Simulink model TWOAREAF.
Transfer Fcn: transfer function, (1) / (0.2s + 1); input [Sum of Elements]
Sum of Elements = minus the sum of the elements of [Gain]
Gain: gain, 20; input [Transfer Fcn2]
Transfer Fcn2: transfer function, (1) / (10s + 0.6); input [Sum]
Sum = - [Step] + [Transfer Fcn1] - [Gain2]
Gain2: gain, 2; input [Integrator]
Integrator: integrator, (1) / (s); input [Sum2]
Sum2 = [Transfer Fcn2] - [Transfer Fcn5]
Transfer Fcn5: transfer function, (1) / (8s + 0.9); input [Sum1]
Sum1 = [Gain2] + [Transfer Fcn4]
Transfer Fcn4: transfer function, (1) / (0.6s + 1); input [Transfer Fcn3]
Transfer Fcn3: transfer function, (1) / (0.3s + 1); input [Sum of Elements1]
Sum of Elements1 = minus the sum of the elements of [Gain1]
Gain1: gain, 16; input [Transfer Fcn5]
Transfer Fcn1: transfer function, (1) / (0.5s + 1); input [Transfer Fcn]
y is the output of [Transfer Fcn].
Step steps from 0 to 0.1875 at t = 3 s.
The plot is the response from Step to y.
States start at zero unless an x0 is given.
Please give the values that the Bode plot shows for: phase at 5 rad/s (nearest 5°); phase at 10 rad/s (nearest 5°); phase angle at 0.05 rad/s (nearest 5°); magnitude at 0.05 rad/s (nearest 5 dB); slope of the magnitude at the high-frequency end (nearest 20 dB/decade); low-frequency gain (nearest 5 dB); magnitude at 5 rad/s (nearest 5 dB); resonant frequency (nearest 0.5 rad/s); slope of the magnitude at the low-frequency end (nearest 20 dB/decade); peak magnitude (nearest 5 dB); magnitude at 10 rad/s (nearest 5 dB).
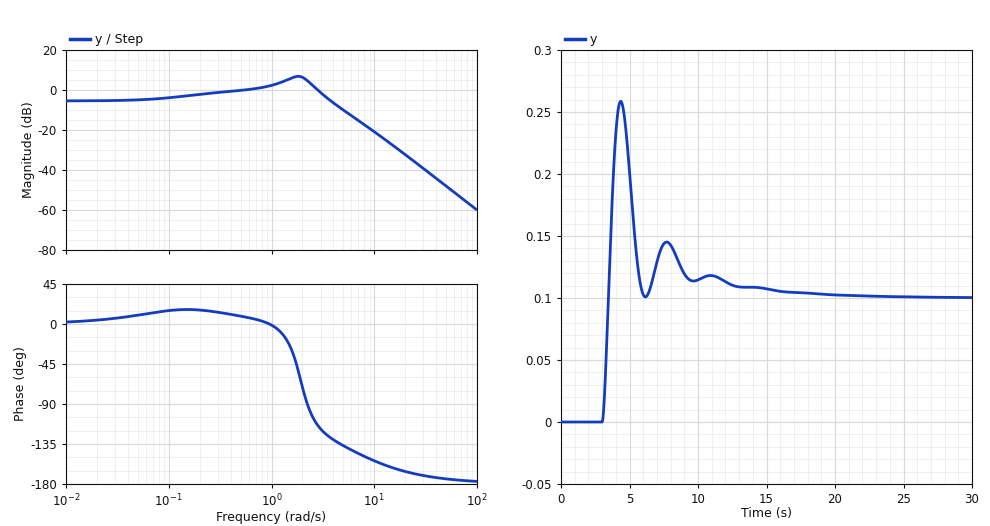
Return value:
-135°
-155°
10°
-5 dB
-40 dB/decade
-5 dB
-10 dB
2.0 rad/s
0 dB/decade
5 dB
-20 dB
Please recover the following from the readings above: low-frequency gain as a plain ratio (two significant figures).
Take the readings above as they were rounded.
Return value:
0.56
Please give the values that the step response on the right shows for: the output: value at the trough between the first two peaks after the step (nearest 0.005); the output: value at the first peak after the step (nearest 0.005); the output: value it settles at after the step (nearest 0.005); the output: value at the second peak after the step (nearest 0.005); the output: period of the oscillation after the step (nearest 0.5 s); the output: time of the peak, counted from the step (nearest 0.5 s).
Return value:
0.100
0.260
0.100
0.145
3.5 s
1.5 s
